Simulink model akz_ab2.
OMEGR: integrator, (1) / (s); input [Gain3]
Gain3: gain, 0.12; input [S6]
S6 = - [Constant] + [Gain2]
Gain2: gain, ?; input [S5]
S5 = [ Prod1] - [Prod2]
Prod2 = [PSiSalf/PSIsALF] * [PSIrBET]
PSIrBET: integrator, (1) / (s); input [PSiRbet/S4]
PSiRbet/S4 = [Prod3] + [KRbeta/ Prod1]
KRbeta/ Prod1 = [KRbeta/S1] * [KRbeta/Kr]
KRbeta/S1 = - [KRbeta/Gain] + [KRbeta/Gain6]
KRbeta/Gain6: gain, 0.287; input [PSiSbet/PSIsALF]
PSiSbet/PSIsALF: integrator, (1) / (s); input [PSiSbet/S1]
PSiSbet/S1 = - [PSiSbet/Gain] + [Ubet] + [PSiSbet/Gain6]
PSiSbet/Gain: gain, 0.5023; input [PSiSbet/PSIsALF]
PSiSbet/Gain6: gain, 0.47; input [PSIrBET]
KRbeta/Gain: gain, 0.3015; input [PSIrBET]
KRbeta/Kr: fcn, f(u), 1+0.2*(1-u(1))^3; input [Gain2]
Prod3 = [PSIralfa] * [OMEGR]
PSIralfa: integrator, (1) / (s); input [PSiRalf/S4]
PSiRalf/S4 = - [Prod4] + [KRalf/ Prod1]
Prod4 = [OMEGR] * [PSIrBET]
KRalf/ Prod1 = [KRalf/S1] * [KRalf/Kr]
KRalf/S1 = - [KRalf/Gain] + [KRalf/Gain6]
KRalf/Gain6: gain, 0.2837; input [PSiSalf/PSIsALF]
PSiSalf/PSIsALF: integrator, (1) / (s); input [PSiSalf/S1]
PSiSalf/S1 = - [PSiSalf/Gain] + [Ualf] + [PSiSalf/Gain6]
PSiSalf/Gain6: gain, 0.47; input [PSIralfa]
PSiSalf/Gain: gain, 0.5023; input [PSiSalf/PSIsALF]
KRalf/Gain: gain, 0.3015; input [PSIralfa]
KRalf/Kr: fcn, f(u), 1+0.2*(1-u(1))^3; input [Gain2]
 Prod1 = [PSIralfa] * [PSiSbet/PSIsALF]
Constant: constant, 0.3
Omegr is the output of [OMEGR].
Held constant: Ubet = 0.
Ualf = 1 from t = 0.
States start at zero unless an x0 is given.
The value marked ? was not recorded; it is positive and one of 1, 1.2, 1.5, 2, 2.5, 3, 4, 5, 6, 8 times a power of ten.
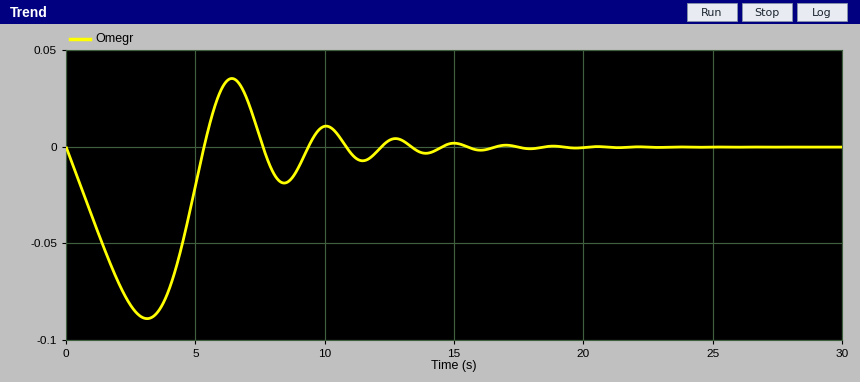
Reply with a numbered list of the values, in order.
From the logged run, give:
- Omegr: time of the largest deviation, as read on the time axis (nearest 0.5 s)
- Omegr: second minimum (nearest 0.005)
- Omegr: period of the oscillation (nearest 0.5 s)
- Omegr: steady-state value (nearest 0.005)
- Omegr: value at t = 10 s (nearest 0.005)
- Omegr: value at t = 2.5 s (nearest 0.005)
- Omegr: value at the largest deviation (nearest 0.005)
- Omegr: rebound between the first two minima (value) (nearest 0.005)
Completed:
1. 3.0 s
2. -0.020
3. 5.5 s
4. 0.000
5. 0.010
6. -0.080
7. -0.090
8. 0.035
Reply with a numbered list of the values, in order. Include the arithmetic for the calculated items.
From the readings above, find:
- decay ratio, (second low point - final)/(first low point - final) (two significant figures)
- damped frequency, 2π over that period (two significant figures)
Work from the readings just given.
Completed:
1. (-0.02 - 0) / (-0.09 - 0) = 0.22
2. 2π / 5.5 = 1.1 rad/s
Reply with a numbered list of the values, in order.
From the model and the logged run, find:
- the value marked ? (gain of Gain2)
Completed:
1. 3
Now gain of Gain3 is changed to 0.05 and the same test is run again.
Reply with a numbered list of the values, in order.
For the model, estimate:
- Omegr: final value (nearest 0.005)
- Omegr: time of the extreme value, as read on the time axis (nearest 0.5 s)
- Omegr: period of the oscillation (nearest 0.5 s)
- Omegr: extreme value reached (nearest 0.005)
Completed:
1. 0.000
2. 4.0 s
3. 7.0 s
4. -0.045
